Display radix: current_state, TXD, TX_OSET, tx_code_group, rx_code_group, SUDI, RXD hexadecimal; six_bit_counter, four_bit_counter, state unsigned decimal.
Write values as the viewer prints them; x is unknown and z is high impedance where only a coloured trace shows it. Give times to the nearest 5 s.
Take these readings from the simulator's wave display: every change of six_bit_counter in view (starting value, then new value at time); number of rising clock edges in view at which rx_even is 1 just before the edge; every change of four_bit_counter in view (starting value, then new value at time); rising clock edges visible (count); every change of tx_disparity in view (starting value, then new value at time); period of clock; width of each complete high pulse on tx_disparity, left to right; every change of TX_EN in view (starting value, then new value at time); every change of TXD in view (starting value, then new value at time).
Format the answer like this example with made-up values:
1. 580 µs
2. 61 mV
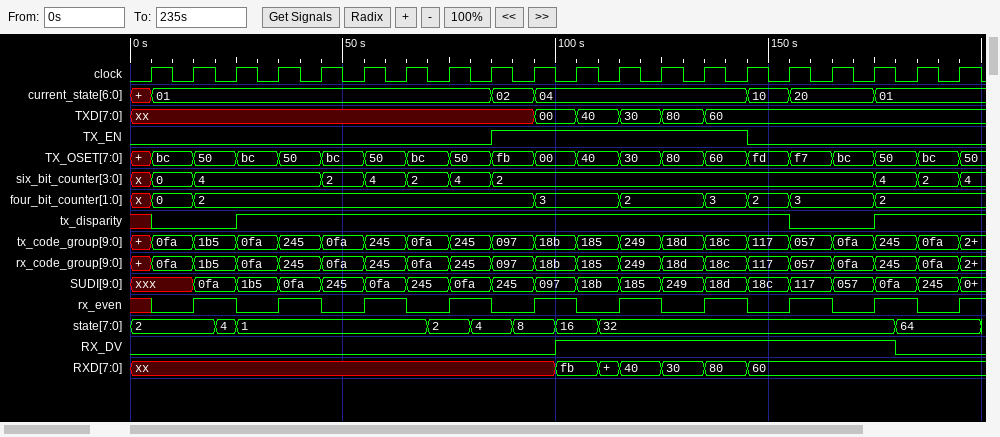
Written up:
1. x, 0 at 5 s, 4 at 15 s, 2 at 45 s, 4 at 55 s, 2 at 65 s, 4 at 75 s, 2 at 85 s, 4 at 175 s, 2 at 185 s, 4 at 195 s
2. 9
3. x, 0 at 5 s, 2 at 15 s, 3 at 95 s, 2 at 115 s, 3 at 135 s, 2 at 145 s, 3 at 155 s, 2 at 175 s
4. 20
5. x, 0 at 5 s, 1 at 25 s, 0 at 155 s, 1 at 175 s
6. 10 s
7. 130 s
8. 0, 1 at 85 s, 0 at 145 s
9. xx, 00 at 95 s, 40 at 105 s, 30 at 115 s, 80 at 125 s, 60 at 135 s
